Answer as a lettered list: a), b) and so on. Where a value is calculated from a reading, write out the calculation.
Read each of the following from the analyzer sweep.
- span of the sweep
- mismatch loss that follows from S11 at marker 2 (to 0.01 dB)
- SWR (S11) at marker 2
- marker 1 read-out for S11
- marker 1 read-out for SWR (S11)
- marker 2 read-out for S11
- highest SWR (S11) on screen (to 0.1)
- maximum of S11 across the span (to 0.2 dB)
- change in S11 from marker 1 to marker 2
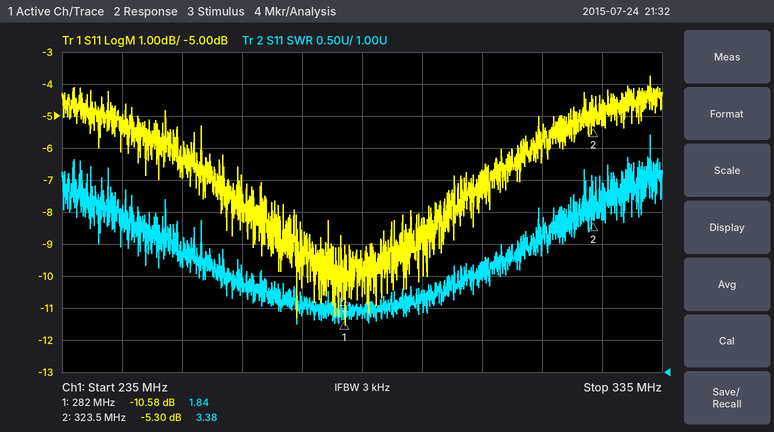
a) 100 MHz
b) −10 log10(1 − 10^(-5.3/10)) ≈ 1.52 dB
c) 3.38
d) -10.58 dB
e) 1.84
f) -5.30 dB
g) 4.7
h) -3.8 dB
i) -5.3 − (-10.58) = 5.28 dB
